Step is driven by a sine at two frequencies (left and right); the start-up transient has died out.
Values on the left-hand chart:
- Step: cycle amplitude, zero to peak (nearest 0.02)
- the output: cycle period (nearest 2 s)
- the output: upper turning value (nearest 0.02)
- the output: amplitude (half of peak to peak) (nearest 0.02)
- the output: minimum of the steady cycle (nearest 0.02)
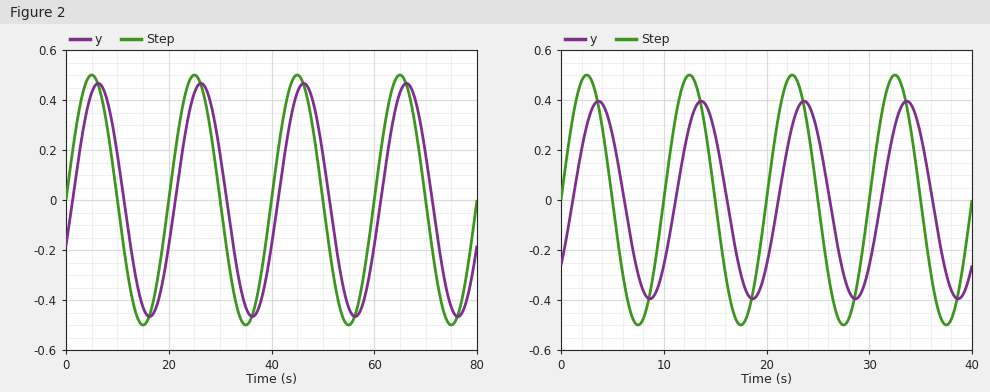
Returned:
0.50
20 s
0.46
0.46
-0.46
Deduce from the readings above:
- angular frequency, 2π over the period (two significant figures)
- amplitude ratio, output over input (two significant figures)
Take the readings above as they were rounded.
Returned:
0.31 rad/s
0.92
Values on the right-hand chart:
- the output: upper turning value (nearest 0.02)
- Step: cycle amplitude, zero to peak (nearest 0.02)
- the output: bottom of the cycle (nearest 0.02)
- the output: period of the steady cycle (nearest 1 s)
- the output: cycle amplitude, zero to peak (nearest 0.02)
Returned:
0.40
0.50
-0.40
10 s
0.40
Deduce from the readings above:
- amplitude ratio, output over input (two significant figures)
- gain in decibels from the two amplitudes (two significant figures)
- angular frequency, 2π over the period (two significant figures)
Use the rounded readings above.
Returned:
0.80
-1.9 dB
0.63 rad/s
